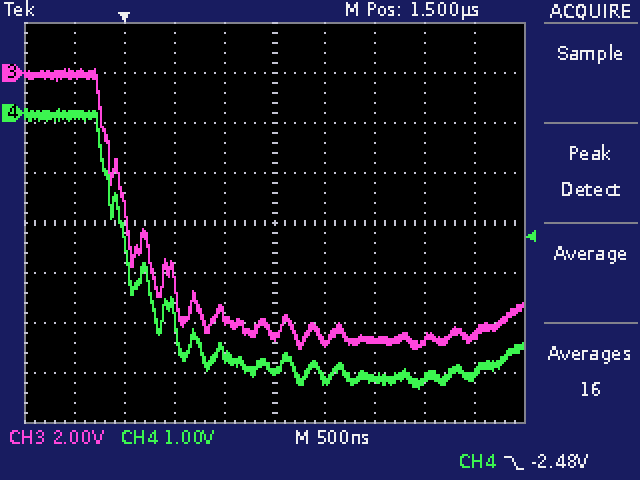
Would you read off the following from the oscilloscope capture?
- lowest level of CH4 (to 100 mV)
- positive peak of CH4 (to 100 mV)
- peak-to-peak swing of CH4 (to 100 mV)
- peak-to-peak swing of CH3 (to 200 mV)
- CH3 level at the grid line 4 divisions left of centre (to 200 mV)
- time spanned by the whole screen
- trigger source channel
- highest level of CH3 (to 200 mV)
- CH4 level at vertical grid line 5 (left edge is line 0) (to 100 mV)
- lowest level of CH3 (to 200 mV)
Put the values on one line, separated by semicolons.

-5.5 V; 100 mV; 5.6 V; 11.2 V; 0.0 V; 5 µs; CH4; 200 mV; -5.2 V; -11.0 V
